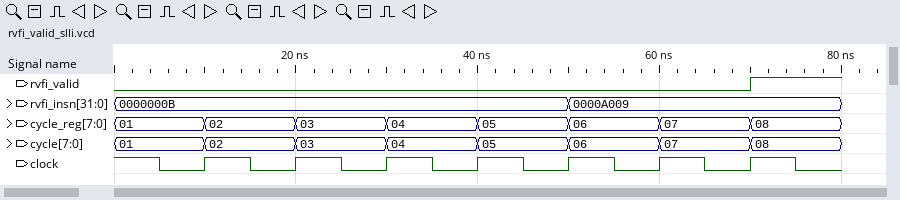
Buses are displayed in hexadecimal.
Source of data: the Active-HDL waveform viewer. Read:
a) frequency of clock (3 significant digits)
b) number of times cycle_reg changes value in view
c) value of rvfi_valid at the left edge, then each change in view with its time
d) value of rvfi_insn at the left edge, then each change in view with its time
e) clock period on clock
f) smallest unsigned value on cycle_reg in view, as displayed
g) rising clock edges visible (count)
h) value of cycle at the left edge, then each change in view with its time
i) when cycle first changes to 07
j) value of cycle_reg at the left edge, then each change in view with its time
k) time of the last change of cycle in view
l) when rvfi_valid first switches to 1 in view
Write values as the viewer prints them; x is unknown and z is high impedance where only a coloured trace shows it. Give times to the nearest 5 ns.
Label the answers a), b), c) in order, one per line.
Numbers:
a) 100 MHz
b) 7
c) 0, 1 at 70 ns
d) 0000000B, 0000A009 at 50 ns
e) 10 ns
f) 01
g) 7
h) 01, 02 at 10 ns, 03 at 20 ns, 04 at 30 ns, 05 at 40 ns, 06 at 50 ns, 07 at 60 ns, 08 at 70 ns
i) 60 ns
j) 01, 02 at 10 ns, 03 at 20 ns, 04 at 30 ns, 05 at 40 ns, 06 at 50 ns, 07 at 60 ns, 08 at 70 ns
k) 70 ns
l) 70 ns
